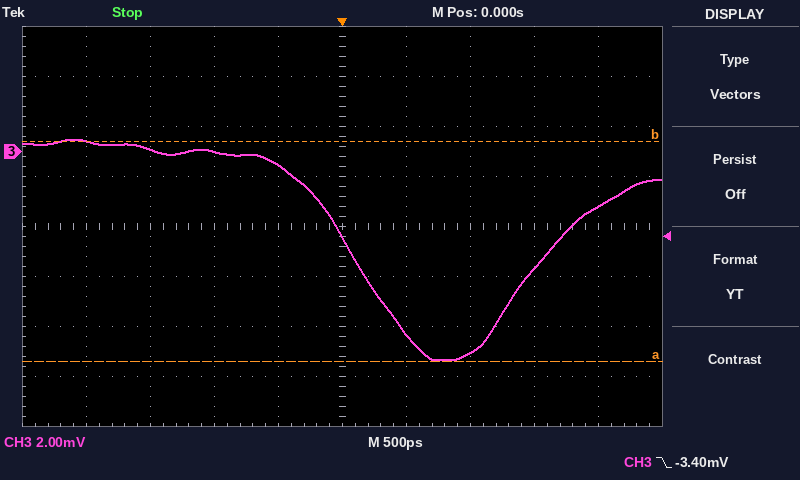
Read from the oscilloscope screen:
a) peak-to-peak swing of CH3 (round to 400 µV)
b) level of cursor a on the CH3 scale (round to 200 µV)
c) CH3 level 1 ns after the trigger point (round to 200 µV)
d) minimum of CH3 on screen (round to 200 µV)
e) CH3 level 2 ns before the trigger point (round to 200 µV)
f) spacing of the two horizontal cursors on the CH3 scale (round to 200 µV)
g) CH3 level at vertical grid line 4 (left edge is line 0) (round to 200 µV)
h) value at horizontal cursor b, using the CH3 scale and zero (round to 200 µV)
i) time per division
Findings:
8.8 mV
-8.4 mV
-8.0 mV
-8.4 mV
400 µV
8.8 mV
-600 µV
400 µV
500 ps
